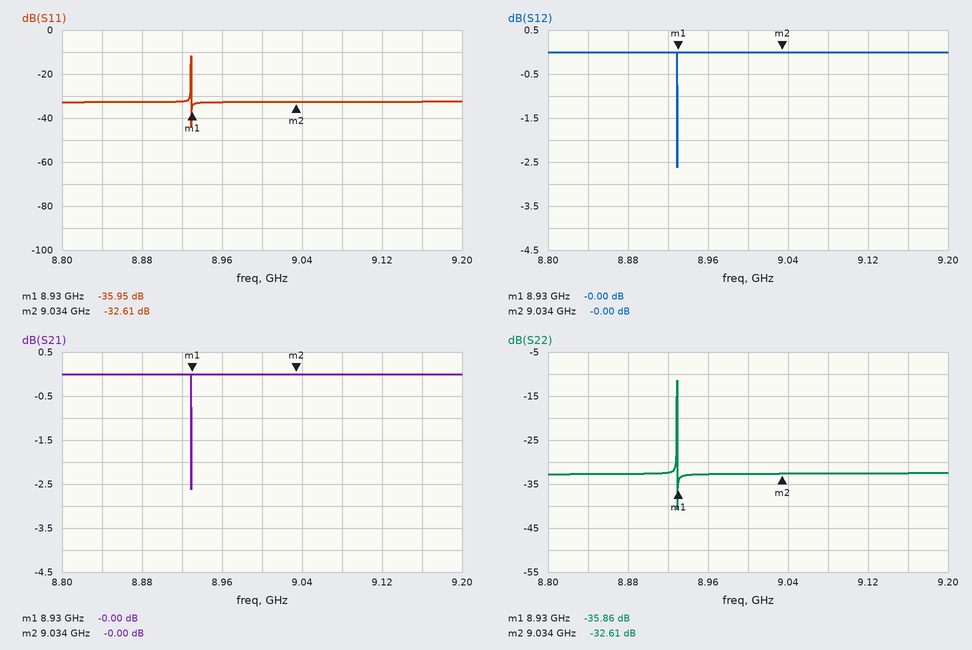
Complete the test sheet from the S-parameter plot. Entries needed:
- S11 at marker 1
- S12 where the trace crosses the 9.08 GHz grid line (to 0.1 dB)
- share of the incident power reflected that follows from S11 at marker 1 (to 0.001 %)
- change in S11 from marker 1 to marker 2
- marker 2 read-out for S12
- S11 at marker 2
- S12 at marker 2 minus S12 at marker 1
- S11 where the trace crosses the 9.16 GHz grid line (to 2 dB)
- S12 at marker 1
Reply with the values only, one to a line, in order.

-35.95 dB
0.0 dB
0.025 %
3.34 dB
-0.00 dB
-32.61 dB
0.00 dB
-32 dB
-0.00 dB
